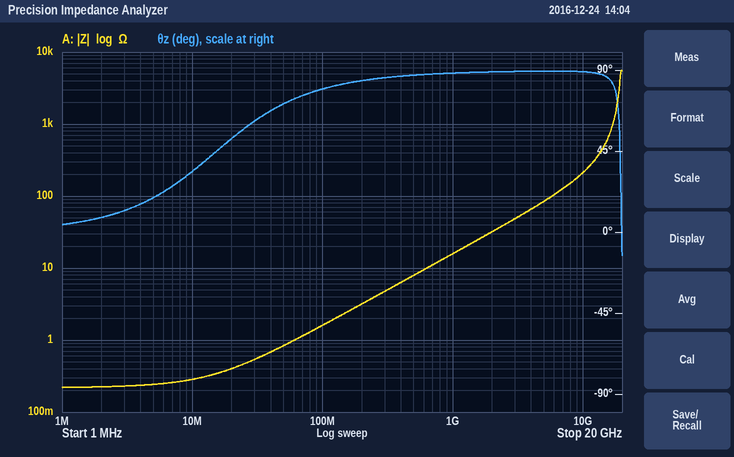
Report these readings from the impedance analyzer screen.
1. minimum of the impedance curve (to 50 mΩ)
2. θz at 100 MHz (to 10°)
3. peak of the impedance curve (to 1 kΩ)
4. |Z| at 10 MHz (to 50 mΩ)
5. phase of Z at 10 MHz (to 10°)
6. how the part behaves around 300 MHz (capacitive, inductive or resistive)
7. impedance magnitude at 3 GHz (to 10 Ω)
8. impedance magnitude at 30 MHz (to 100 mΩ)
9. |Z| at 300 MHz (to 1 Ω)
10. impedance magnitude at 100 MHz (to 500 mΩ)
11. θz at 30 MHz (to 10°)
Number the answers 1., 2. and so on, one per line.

1. 200 mΩ
2. 80°
3. 6 kΩ
4. 300 mΩ
5. 30°
6. inductive
7. 50 Ω
8. 500 mΩ
9. 5 Ω
10. 1.5 Ω
11. 60°
